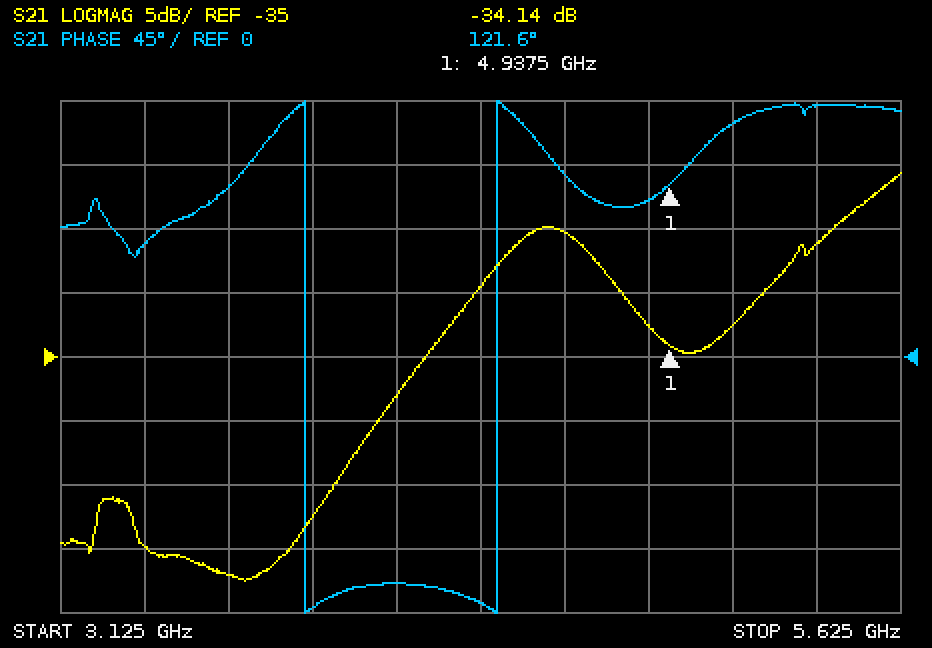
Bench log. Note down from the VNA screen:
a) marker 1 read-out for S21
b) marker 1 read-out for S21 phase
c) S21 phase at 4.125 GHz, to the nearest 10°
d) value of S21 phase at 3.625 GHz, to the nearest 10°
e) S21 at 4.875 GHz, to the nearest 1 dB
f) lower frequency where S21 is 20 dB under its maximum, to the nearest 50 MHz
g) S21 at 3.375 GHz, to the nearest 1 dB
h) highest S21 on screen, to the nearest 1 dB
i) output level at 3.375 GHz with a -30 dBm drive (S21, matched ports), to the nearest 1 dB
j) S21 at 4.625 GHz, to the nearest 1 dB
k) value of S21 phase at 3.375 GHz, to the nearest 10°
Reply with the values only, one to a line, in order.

-34.14 dB
121.6°
-160°
120°
-33 dB
4.05 GHz
-50 dB
-21 dB
-80 dBm
-25 dB
80°
